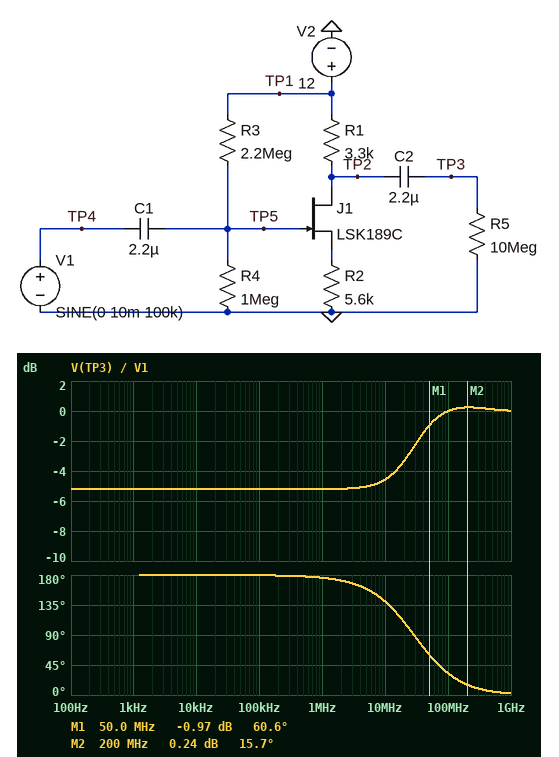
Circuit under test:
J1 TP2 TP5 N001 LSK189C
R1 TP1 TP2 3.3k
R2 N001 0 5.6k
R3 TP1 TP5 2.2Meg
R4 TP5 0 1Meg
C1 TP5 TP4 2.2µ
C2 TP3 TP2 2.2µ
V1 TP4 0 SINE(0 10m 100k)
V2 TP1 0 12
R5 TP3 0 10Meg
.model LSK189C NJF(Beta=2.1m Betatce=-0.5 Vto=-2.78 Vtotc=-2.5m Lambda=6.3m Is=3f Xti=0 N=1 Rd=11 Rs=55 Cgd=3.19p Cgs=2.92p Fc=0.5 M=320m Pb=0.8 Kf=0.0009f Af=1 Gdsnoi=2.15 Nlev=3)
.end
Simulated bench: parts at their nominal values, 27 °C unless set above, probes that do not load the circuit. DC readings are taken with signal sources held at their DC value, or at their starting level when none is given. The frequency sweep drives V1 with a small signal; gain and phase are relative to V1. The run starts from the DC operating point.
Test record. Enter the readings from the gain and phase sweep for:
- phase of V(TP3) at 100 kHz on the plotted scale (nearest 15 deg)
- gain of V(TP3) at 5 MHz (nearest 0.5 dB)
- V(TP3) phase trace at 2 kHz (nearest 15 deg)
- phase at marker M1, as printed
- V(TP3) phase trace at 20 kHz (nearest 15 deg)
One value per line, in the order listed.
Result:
180 deg
-5.0 dB
180 deg
60.6 deg
180 deg
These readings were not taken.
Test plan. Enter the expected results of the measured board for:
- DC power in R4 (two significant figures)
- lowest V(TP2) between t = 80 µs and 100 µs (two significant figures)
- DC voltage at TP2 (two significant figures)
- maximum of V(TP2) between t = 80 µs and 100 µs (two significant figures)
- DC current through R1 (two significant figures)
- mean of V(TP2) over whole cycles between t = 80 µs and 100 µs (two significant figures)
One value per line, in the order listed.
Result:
14 µW
8.6 V
8.6 V
8.6 V
1.0 mA
8.6 V
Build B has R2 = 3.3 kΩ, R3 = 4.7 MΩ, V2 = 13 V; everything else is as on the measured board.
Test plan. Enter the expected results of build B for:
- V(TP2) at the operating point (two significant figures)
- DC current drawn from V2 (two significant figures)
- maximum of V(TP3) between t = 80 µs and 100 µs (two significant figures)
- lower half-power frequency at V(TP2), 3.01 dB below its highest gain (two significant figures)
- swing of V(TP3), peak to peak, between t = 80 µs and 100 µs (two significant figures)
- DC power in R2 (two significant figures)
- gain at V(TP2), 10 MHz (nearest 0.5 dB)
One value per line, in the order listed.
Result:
8.8 V
1.3 mA
9.0 mV
140 mHz
18 mV
5.4 mW
-1.0 dB
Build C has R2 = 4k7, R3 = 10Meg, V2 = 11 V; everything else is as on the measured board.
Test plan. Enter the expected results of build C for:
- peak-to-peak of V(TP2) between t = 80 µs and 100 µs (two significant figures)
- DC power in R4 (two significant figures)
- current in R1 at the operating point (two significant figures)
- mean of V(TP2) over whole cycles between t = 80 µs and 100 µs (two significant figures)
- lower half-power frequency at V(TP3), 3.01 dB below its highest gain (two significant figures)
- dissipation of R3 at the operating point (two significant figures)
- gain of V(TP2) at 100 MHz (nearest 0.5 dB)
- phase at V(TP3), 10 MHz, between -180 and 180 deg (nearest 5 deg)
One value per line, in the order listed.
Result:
13 mV
1.0 µW
680 µA
8.8 V
23 MHz
10 µW
0 dB
150 deg
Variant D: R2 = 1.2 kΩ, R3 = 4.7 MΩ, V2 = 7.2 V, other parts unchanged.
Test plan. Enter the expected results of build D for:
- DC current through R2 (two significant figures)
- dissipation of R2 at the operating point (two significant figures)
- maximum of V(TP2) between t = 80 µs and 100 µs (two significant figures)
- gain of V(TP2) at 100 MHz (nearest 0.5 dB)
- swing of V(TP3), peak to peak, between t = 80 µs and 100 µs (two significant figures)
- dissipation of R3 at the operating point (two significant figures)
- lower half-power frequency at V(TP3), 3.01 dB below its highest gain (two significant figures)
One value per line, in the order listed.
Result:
1.5 mA
2.8 mW
2.1 V
-0.5 dB
1.3 mV
7.5 µW
38 MHz
